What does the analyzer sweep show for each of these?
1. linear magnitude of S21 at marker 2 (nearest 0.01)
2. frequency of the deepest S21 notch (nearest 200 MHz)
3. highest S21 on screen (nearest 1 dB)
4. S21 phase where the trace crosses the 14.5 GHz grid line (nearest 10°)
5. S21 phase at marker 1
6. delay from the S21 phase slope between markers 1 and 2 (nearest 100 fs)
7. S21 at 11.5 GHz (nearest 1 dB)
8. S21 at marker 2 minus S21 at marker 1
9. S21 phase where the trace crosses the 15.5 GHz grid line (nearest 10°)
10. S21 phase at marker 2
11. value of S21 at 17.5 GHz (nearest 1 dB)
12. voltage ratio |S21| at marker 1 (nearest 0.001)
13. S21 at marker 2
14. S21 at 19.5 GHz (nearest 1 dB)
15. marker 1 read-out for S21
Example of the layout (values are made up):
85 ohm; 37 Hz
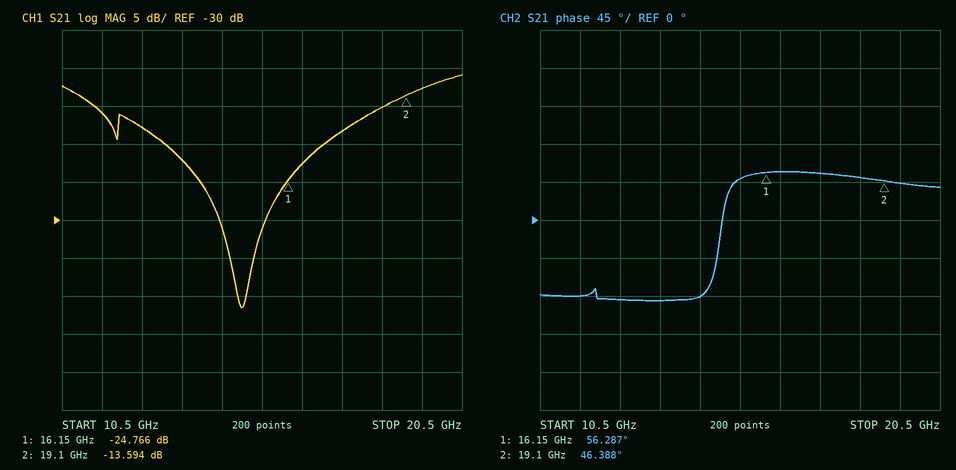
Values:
0.21; 15.0 GHz; -11 dB; -90°; 56.287°; 9.3 ps; -16 dB; 11.172 dB; 50°; 46.388°; -18 dB; 0.058; -13.594 dB; -13 dB; -24.766 dB
